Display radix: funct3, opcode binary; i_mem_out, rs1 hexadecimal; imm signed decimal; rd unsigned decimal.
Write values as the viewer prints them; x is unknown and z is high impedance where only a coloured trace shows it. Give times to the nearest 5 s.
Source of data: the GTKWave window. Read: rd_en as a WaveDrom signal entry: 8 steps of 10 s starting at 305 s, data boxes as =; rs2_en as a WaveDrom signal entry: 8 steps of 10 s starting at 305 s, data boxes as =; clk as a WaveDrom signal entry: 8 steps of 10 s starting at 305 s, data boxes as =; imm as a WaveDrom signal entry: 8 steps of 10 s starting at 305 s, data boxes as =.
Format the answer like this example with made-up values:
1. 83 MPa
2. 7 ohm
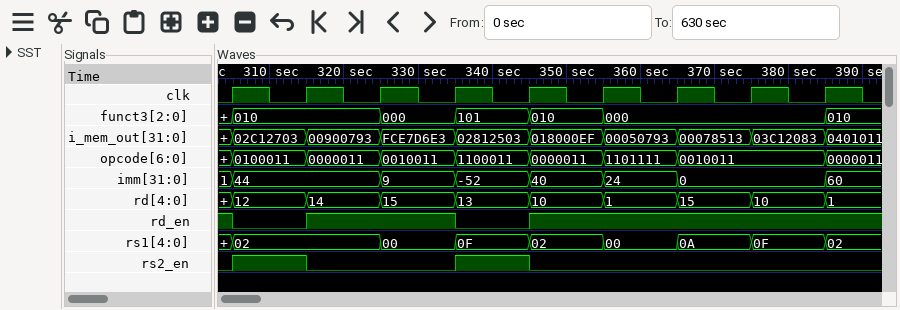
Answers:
1. {name: 'rd_en', wave: '01.01...'}
2. {name: 'rs2_en', wave: '10.10...'}
3. {name: 'clk', wave: 'p.......'}
4. {name: 'imm', wave: '=.=====.', data: '44 9 -52 40 24 0'}
